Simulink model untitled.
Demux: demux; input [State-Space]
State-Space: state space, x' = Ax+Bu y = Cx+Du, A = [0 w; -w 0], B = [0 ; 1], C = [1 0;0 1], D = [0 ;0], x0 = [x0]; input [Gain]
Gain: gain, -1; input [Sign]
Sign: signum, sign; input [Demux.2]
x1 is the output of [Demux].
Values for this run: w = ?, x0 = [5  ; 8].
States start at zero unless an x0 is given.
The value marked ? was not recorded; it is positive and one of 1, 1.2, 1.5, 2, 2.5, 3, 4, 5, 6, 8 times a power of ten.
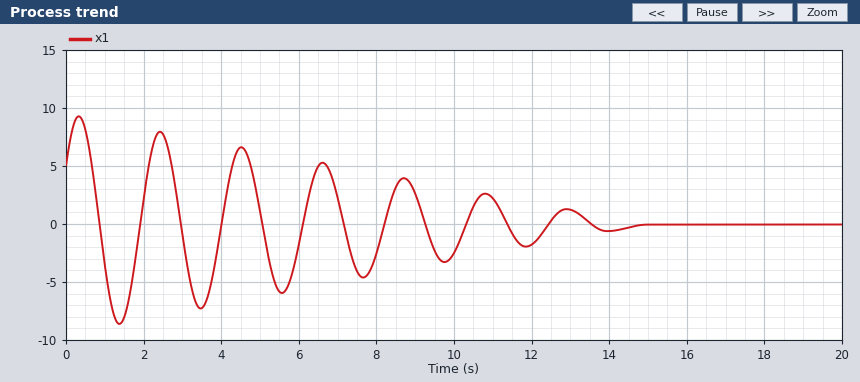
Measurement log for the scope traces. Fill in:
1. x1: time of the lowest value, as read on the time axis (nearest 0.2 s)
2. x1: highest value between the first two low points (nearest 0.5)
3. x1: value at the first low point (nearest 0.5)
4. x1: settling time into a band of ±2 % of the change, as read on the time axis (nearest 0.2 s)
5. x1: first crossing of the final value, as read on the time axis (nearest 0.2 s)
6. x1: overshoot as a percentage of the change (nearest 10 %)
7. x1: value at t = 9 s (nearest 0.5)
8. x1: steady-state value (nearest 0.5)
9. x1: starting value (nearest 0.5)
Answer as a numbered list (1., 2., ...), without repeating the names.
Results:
1. 1.4 s
2. 8.0
3. -8.5
4. 14.8 s
5. 0.8 s
6. 170 %
7. 2.5
8. 0.0
9. 5.0
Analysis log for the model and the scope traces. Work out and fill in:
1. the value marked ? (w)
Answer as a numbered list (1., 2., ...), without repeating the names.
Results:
1. 3
